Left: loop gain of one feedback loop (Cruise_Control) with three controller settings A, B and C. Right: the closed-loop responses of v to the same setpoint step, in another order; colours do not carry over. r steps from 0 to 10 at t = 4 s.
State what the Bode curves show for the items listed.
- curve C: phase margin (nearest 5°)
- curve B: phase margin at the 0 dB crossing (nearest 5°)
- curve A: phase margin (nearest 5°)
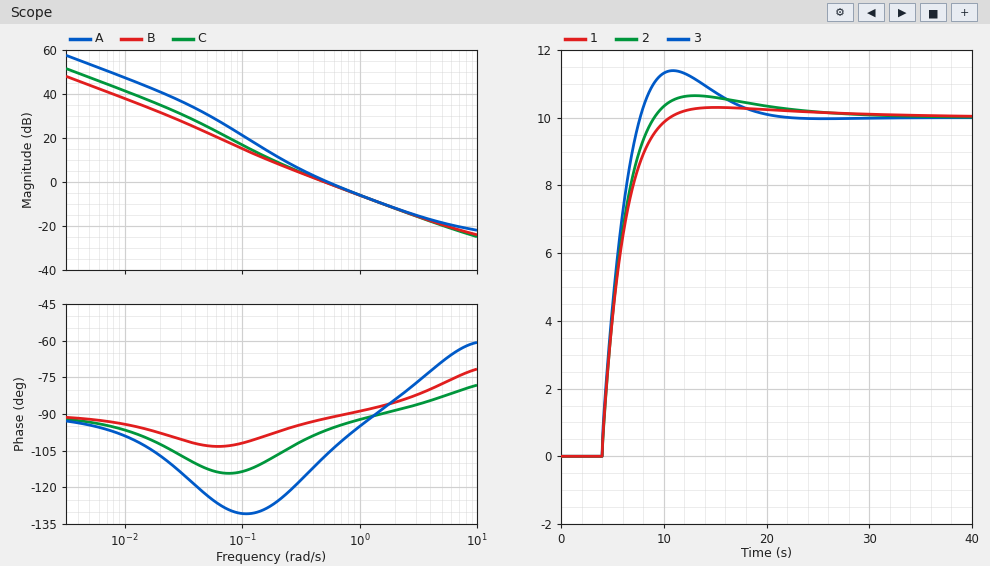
85°
90°
75°
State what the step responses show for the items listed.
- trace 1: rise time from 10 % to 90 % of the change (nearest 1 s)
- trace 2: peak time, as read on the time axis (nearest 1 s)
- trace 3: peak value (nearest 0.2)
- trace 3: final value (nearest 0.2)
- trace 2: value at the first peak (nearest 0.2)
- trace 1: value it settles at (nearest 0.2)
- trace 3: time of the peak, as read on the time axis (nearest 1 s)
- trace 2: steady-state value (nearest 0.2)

4 s
13 s
11.4
10.0
10.6
10.0
11 s
10.0
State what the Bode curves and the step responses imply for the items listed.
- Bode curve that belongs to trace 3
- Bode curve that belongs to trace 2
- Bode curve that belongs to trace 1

A
C
B
